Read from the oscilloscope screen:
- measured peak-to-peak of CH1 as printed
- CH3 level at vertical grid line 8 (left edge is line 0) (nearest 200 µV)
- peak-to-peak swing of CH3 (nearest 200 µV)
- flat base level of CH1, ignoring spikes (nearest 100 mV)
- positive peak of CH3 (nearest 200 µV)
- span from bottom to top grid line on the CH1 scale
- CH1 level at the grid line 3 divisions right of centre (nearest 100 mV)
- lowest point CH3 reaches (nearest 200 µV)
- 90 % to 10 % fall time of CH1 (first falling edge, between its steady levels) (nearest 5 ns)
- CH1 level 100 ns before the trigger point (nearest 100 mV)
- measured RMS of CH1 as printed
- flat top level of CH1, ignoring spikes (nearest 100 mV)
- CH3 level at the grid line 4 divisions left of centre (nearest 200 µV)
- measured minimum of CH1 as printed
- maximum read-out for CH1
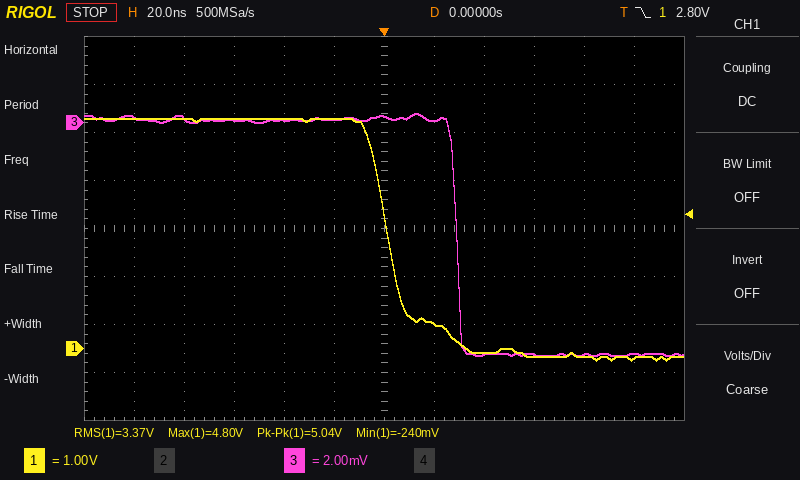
5.04 V
-9.6 mV
10.0 mV
-200 mV
400 µV
8 V
-200 mV
-9.6 mV
30 ns
4.8 V
3.37 V
4.8 V
200 µV
-240 mV
4.80 V
